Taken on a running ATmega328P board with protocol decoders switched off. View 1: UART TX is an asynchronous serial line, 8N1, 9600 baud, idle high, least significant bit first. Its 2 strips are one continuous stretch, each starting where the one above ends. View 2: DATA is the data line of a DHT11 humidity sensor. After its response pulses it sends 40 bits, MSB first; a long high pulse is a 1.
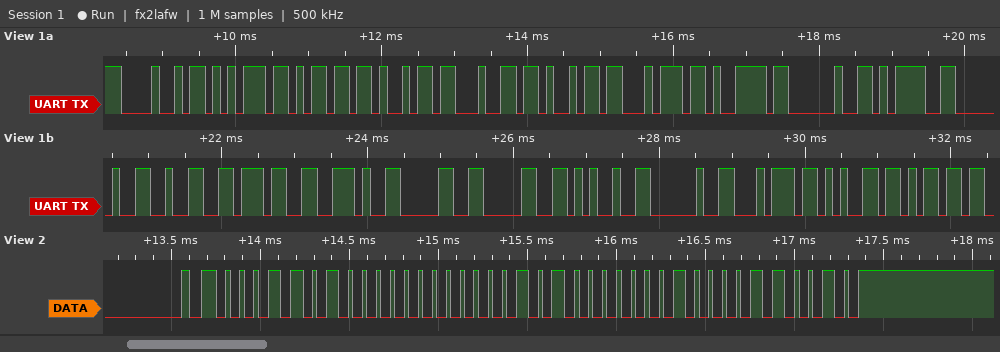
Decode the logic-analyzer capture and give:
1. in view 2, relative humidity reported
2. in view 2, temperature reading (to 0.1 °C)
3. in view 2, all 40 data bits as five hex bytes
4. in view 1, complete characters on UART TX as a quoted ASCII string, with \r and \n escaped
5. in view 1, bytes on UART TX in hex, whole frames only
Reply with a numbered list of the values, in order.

1. 26 %
2. 20.4 °C
3. 1A 00 14 04 32
4. "Humidity = 27.00% tem"
5. 48 75 6D 69 64 69 74 79 20 3D 20 32 37 2E 30 30 25 20 74 65 6D
